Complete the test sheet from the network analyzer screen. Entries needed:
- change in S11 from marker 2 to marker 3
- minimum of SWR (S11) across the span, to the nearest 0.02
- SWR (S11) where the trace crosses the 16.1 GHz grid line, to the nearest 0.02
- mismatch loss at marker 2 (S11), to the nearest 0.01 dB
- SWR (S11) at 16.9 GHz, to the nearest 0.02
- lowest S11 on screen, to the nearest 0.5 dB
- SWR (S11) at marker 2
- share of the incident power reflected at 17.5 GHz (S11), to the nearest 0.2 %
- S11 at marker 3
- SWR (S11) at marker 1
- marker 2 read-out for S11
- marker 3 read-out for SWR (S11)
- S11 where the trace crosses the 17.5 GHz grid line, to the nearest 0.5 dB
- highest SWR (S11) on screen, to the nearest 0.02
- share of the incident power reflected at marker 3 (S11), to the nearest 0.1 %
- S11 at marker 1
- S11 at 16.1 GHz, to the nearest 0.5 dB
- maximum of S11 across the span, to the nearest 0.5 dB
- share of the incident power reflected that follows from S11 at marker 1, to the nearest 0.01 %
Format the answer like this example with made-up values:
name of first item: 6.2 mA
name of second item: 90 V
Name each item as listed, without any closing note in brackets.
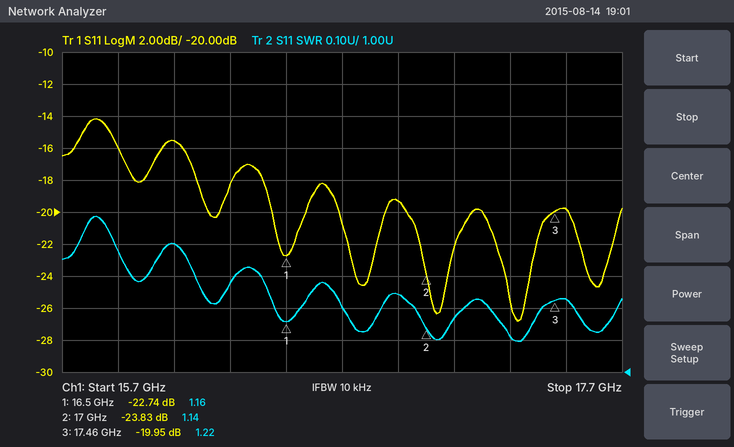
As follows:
change in S11 from marker 2 to marker 3: 3.88 dB
minimum of SWR (S11) across the span, to the nearest 0.02: 1.10
SWR (S11) where the trace crosses the 16.1 GHz grid line, to the nearest 0.02: 1.40
mismatch loss at marker 2 (S11), to the nearest 0.01 dB: 0.02 dB
SWR (S11) at 16.9 GHz, to the nearest 0.02: 1.24
lowest S11 on screen, to the nearest 0.5 dB: -27.0 dB
SWR (S11) at marker 2: 1.14
share of the incident power reflected at 17.5 GHz (S11), to the nearest 0.2 %: 1.0 %
S11 at marker 3: -19.95 dB
SWR (S11) at marker 1: 1.16
marker 2 read-out for S11: -23.83 dB
marker 3 read-out for SWR: 1.22
S11 where the trace crosses the 17.5 GHz grid line, to the nearest 0.5 dB: -20.0 dB
highest SWR (S11) on screen, to the nearest 0.02: 1.48
share of the incident power reflected at marker 3 (S11), to the nearest 0.1 %: 1.0 %
S11 at marker 1: -22.74 dB
S11 at 16.1 GHz, to the nearest 0.5 dB: -15.5 dB
maximum of S11 across the span, to the nearest 0.5 dB: -14.0 dB
share of the incident power reflected that follows from S11 at marker 1, to the nearest 0.01 %: 0.53 %
